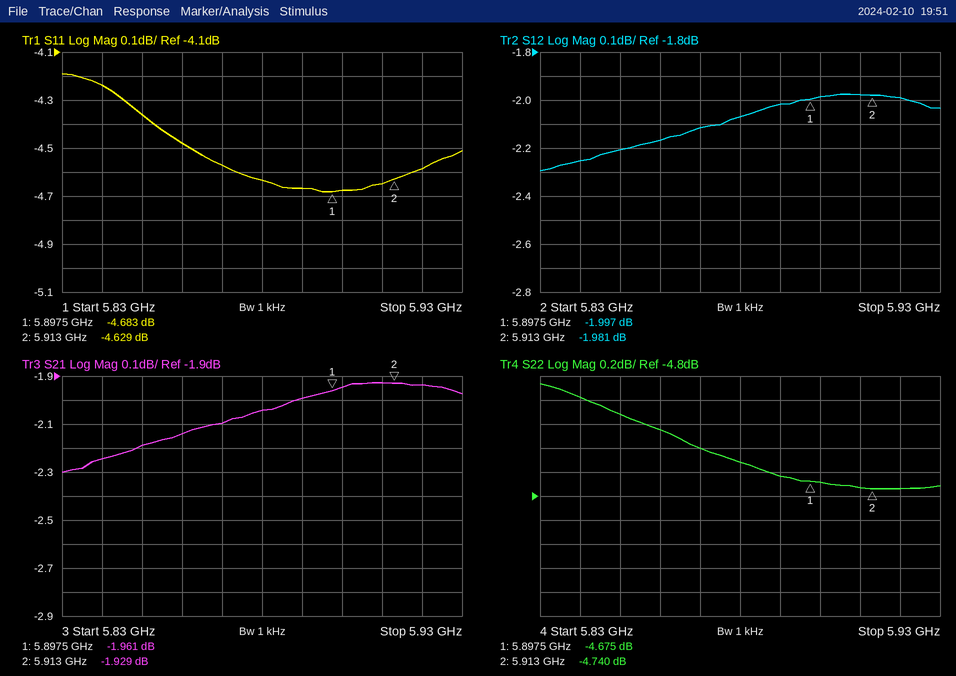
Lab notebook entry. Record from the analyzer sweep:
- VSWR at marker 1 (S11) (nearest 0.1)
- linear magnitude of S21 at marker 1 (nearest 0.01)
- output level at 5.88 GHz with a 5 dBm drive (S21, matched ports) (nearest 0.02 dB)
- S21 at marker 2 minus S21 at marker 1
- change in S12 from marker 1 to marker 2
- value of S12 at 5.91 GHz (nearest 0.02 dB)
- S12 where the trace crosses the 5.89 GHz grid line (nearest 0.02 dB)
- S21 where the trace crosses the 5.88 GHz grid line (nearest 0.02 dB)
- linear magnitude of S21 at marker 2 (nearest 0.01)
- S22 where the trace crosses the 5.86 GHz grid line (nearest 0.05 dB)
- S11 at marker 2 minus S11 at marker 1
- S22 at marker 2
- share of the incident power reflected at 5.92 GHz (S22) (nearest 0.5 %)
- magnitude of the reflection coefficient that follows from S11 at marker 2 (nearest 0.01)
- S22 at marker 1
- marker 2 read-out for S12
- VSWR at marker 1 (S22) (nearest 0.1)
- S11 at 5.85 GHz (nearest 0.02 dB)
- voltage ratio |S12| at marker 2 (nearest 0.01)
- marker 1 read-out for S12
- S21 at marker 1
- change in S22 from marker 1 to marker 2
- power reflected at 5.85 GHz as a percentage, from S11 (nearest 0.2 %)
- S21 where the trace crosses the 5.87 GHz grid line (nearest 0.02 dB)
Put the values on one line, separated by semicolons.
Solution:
3.8; 0.80; 2.96 dBm; 0.032 dB; 0.016 dB; -1.98 dB; -2.02 dB; -2.04 dB; 0.80; -4.25 dB; 0.054 dB; -4.740 dB; 33.5 %; 0.59; -4.675 dB; -1.981 dB; 3.8; -4.36 dB; 0.80; -1.997 dB; -1.961 dB; -0.065 dB; 36.6 %; -2.10 dB
